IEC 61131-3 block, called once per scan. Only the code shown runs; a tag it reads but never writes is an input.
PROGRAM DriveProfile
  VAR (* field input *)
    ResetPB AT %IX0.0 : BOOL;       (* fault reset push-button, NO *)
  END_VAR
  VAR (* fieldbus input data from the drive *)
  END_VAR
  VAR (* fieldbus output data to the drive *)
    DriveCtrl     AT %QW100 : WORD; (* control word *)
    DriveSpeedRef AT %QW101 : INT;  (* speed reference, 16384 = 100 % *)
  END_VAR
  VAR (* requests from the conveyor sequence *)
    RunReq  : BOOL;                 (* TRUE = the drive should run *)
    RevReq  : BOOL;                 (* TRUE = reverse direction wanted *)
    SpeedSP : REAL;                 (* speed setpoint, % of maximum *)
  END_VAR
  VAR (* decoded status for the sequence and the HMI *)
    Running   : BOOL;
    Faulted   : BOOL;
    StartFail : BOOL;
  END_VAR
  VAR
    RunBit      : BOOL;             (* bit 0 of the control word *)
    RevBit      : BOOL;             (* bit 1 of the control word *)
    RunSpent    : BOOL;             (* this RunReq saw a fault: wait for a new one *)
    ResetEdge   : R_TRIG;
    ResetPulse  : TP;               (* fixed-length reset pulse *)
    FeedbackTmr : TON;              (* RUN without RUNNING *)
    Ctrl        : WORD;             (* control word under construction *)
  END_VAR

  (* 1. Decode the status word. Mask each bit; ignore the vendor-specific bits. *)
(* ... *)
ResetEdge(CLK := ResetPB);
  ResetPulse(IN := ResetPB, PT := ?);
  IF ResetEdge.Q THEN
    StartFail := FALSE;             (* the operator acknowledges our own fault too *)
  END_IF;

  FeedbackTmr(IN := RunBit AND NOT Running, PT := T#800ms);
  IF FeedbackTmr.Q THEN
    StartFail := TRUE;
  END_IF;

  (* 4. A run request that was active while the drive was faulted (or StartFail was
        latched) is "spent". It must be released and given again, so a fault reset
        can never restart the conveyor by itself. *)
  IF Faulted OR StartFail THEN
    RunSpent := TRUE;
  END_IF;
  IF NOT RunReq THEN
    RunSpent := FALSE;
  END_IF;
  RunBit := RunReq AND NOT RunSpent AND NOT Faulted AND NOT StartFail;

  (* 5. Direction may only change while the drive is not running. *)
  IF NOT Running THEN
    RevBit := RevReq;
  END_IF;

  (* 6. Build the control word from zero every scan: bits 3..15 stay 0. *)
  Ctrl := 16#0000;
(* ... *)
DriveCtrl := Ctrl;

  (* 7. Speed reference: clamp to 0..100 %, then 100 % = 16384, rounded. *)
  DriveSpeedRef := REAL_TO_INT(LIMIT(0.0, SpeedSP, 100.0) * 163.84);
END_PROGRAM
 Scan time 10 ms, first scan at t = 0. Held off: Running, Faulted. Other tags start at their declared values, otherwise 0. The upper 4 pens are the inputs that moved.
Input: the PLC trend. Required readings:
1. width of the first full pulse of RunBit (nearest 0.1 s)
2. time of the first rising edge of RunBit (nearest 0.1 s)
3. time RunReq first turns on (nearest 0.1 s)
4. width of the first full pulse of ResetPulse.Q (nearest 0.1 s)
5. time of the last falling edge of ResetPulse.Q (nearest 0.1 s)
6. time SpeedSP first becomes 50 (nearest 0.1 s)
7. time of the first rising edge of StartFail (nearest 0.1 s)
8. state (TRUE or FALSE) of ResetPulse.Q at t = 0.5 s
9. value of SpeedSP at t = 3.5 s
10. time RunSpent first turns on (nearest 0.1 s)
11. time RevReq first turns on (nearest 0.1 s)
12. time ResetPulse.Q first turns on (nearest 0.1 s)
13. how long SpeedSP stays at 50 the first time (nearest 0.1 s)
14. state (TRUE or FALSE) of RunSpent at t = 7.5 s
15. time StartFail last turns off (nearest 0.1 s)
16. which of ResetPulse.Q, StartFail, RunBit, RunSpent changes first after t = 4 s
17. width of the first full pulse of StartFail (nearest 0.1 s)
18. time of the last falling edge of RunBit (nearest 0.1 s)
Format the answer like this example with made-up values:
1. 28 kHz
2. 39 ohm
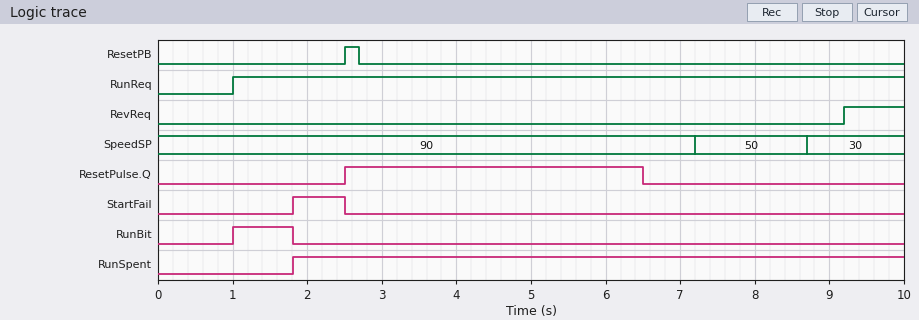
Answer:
1. 0.8 s
2. 1.0 s
3. 1.0 s
4. 4.0 s
5. 6.5 s
6. 7.2 s
7. 1.8 s
8. FALSE
9. 90
10. 1.8 s
11. 9.2 s
12. 2.5 s
13. 1.5 s
14. TRUE
15. 2.5 s
16. ResetPulse.Q
17. 0.7 s
18. 1.8 s
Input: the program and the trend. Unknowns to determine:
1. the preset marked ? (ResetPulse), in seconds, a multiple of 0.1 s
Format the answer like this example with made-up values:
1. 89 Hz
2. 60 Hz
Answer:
1. 4.0 s
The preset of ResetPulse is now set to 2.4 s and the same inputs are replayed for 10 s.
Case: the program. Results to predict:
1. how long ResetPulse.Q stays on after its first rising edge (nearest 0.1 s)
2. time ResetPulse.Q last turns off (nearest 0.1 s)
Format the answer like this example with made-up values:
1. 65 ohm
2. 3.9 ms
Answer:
1. 2.4 s
2. 4.9 s
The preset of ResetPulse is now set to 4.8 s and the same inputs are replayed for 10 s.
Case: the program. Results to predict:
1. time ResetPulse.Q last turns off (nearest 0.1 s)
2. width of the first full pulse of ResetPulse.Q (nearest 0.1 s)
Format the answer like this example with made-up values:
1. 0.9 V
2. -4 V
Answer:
1. 7.3 s
2. 4.8 s
